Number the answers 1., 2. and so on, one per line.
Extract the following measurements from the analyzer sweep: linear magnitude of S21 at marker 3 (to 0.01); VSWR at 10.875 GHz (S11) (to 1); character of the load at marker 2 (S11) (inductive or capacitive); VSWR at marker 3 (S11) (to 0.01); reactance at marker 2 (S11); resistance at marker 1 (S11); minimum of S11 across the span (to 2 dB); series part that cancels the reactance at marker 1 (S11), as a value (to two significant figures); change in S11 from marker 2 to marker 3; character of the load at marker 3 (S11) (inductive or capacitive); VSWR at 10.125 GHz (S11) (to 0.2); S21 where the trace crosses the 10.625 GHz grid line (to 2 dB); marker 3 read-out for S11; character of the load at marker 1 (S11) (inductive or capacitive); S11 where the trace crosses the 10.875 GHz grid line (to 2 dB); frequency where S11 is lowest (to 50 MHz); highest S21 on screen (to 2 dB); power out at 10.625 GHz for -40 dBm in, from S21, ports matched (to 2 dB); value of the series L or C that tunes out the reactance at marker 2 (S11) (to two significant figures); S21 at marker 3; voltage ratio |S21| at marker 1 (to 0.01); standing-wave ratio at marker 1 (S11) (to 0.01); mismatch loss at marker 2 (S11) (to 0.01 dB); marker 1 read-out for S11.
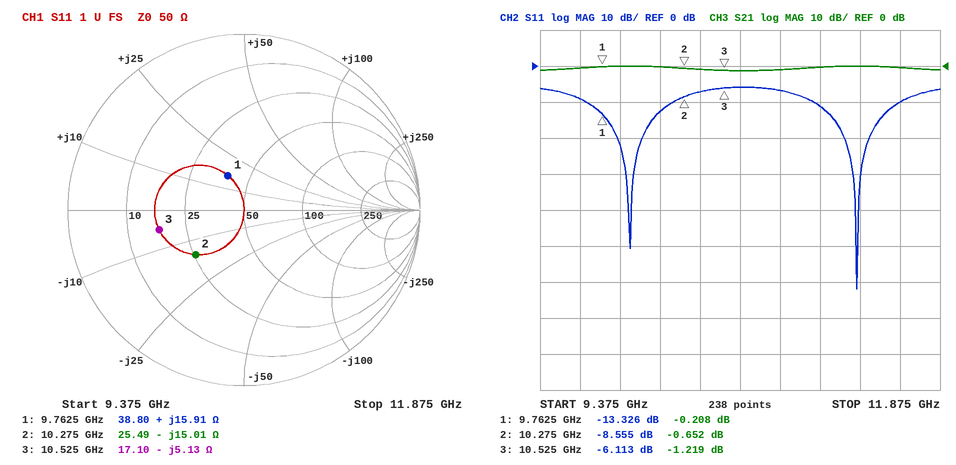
1. 0.87
2. 3
3. capacitive
4. 2.96
5. -15.01 Ω
6. 38.80 Ω
7. -62 dB
8. 1.0 pF
9. 2.442 dB
10. capacitive
11. 1.6
12. -2 dB
13. -6.113 dB
14. inductive
15. -6 dB
16. 11.35 GHz
17. 0 dB
18. -42 dBm
19. 230 pH
20. -1.219 dB
21. 0.98
22. 1.55
23. 0.65 dB
24. -13.326 dB
